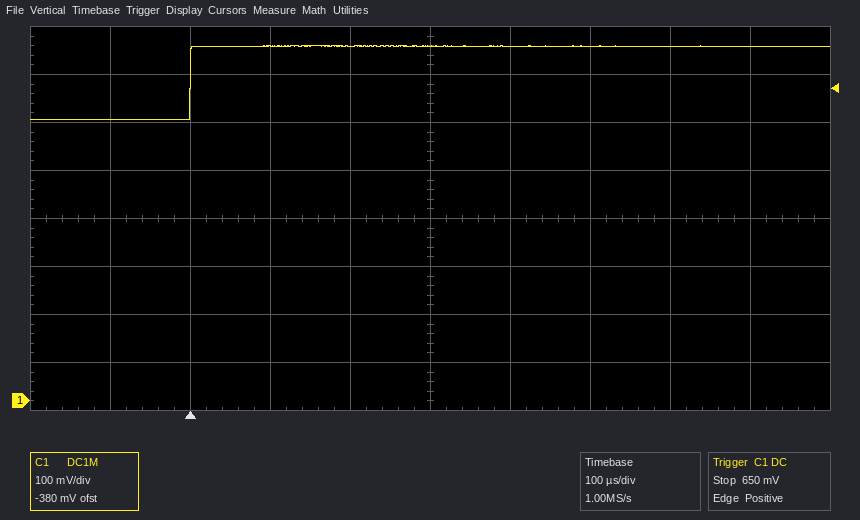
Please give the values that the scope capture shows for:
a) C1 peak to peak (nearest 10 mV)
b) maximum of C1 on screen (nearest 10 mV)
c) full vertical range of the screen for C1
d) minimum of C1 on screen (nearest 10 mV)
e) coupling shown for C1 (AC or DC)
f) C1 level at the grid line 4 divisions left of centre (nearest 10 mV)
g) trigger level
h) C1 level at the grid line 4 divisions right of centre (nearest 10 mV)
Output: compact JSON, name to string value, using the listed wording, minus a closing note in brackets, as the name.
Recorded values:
{"C1 peak to peak": "150 mV", "maximum of C1 on screen": "740 mV", "full vertical range of the screen for C1": "800 mV", "minimum of C1 on screen": "590 mV", "coupling shown for C1": "DC", "C1 level at the grid line 4 divisions left of centre": "590 mV", "trigger level": "650 mV", "C1 level at the grid line 4 divisions right of centre": "740 mV"}
